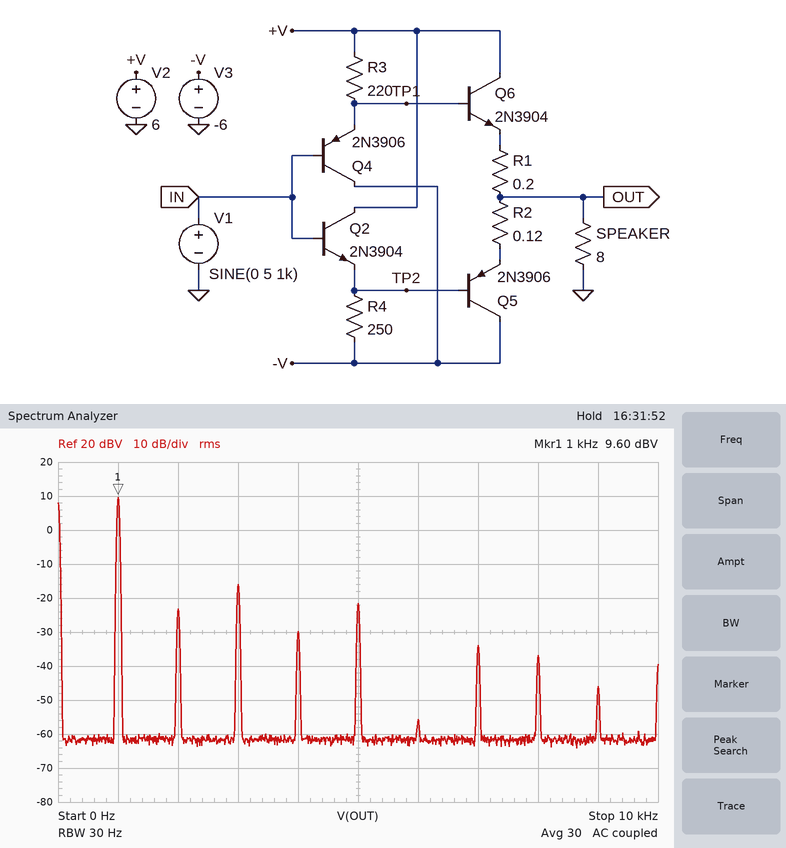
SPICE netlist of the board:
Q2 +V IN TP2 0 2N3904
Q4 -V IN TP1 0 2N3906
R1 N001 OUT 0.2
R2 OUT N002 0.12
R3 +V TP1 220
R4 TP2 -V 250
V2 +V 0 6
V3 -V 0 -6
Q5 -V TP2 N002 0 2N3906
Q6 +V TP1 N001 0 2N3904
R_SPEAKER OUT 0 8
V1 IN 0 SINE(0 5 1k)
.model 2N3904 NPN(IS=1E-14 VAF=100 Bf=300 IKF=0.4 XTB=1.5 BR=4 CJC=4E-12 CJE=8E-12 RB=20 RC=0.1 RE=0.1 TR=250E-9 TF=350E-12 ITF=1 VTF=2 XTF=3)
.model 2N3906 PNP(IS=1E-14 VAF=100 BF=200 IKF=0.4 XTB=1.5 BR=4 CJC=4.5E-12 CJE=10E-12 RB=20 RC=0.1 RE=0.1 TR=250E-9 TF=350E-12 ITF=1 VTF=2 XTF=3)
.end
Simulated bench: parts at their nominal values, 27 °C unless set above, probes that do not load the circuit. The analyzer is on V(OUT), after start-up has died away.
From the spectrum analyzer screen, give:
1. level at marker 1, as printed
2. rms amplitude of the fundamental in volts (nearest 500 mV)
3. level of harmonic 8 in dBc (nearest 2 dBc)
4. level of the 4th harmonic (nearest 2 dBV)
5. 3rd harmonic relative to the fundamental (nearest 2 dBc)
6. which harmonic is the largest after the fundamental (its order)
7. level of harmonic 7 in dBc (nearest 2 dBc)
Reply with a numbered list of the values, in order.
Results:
1. 9.60 dBV
2. 3.0 V
3. -46 dBc
4. -30 dBV
5. -26 dBc
6. 3
7. -44 dBc
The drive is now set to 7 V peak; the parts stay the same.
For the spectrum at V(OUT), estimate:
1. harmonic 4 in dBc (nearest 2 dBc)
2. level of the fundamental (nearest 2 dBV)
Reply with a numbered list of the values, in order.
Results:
1. -44 dBc
2. 10 dBV
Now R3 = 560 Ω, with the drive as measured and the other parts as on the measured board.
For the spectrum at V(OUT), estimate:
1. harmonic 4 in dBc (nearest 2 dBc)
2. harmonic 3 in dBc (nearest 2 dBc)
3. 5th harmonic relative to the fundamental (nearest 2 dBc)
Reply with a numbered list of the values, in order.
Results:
1. -46 dBc
2. -22 dBc
3. -30 dBc
